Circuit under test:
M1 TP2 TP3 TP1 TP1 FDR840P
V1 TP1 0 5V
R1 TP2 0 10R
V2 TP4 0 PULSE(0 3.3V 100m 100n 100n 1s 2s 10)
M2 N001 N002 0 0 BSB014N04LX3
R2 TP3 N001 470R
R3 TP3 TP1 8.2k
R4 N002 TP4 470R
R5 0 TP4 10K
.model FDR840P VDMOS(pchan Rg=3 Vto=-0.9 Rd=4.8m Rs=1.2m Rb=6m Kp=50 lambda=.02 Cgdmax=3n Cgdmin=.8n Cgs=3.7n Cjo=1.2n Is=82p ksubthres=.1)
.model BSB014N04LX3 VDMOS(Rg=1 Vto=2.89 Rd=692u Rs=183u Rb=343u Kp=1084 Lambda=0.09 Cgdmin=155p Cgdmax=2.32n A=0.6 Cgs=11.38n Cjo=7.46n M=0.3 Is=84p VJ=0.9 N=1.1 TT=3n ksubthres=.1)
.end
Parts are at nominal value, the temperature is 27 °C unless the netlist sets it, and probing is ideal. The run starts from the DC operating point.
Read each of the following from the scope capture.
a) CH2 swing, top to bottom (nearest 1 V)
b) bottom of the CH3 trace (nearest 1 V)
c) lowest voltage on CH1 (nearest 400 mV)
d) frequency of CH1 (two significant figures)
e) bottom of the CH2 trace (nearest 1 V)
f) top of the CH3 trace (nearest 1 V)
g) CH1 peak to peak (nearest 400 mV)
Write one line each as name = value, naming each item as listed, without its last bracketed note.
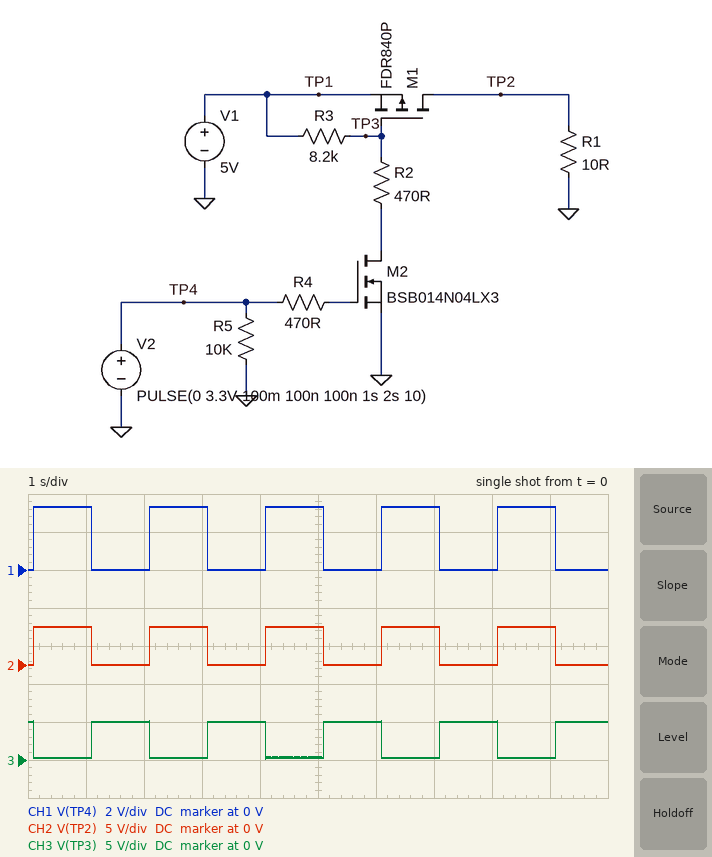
CH2 swing, top to bottom = 5 V
bottom of the CH3 trace = 0 V
lowest voltage on CH1 = 0 V
frequency of CH1 = 500 mHz
bottom of the CH2 trace = 0 V
top of the CH3 trace = 5 V
CH1 peak to peak = 3.2 V
